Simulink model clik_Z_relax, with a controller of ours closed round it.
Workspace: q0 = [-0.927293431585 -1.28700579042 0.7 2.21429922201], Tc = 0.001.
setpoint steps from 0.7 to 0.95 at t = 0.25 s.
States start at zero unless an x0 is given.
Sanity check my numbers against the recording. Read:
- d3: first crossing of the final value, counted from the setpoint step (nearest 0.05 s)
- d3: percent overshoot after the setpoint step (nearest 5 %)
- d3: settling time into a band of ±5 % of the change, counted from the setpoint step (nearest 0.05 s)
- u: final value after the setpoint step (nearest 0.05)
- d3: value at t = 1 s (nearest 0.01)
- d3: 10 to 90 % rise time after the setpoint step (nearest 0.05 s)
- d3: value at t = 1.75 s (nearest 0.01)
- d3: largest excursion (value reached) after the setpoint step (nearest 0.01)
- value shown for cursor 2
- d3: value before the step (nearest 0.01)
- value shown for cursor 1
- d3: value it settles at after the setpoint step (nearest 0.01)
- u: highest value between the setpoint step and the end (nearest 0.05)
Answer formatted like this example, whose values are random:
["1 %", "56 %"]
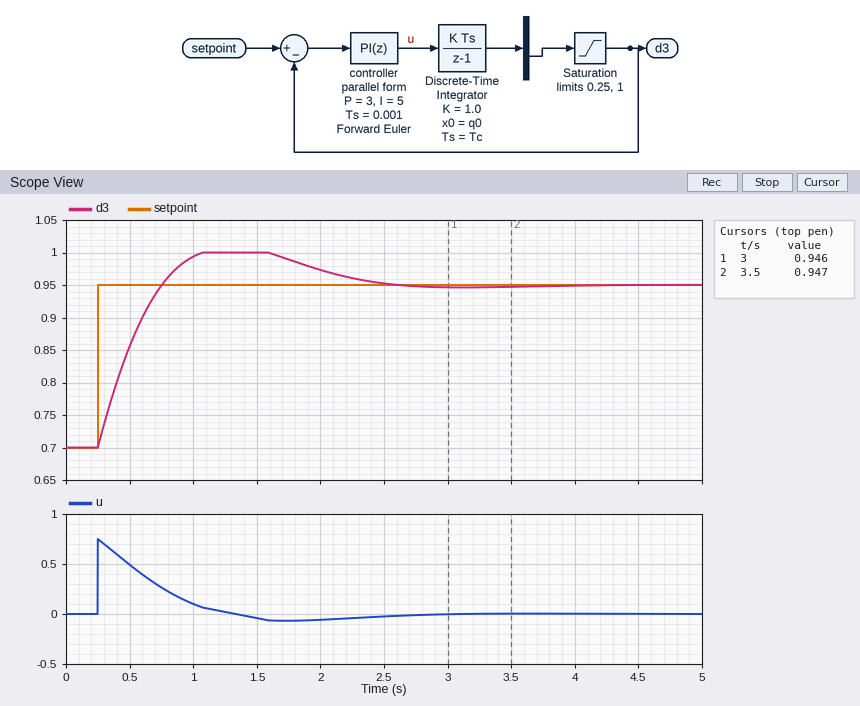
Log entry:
["0.50 s", "20 %", "1.95 s", "0.00", "0.99", "0.40 s", "0.99", "1.00", "0.947", "0.70", "0.946", "0.95", "0.75"]
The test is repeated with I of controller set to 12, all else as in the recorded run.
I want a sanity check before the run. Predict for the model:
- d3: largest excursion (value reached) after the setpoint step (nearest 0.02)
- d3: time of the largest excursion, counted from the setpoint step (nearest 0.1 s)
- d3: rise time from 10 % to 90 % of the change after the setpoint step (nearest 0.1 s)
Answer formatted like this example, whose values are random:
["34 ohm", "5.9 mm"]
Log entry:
["1.00", "0.5 s", "0.3 s"]
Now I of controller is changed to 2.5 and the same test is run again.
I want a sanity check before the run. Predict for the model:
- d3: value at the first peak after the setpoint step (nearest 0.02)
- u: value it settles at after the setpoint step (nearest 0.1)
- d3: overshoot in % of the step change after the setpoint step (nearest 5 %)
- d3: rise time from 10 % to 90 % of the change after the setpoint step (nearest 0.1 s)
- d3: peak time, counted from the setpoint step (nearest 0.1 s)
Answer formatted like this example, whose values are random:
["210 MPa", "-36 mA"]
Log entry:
["0.98", "0.0", "15 %", "0.5 s", "1.3 s"]
